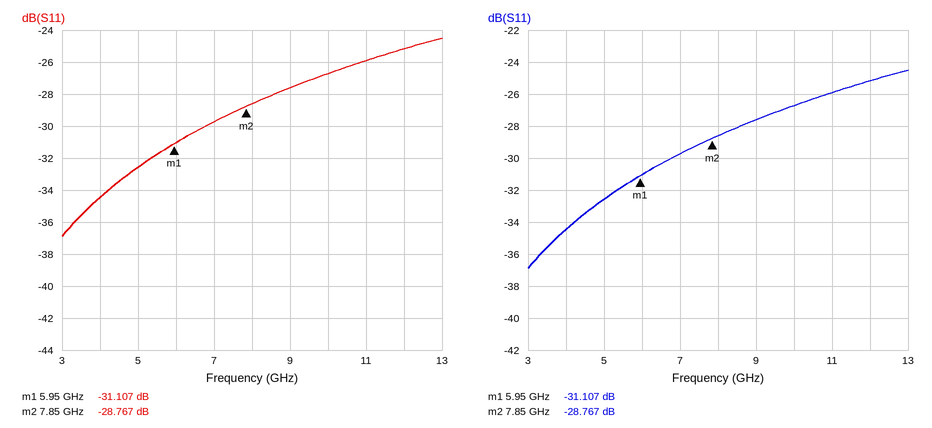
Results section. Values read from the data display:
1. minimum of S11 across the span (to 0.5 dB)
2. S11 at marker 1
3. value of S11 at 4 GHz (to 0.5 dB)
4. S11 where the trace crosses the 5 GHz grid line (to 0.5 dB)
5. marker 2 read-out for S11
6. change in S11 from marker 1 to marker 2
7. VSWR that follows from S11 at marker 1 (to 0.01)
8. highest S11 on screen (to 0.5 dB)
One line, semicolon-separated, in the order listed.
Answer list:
-37.0 dB; -31.107 dB; -34.5 dB; -32.5 dB; -28.767 dB; 2.340 dB; 1.06; -24.5 dB
